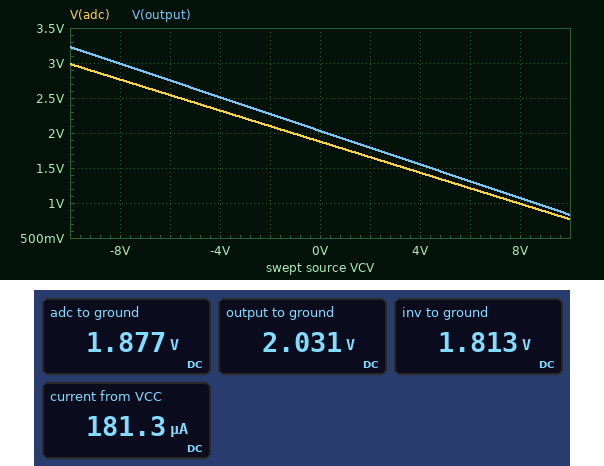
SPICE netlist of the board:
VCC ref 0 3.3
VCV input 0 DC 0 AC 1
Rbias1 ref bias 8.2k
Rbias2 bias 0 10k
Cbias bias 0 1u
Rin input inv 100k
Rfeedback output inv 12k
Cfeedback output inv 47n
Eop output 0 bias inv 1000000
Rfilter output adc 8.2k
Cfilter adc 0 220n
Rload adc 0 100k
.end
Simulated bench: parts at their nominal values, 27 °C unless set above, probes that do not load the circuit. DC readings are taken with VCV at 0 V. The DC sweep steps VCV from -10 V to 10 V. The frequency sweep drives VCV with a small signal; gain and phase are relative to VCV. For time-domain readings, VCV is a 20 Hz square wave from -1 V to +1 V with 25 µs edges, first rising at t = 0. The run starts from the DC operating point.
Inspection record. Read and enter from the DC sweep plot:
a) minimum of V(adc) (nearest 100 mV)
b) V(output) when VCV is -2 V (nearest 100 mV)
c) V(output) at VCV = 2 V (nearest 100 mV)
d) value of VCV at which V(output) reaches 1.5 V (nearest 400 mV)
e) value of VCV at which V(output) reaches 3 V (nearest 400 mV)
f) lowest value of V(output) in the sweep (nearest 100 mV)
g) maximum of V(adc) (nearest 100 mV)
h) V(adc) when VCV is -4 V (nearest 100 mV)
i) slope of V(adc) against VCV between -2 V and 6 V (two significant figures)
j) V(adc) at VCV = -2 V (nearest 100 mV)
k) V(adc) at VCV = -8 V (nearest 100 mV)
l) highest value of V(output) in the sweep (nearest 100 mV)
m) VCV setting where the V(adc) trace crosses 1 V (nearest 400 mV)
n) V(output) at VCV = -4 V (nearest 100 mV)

800 mV
2.3 V
1.8 V
4.4 V
-8.0 V
800 mV
3.0 V
2.3 V
-0.11 V/V
2.1 V
2.8 V
3.2 V
8.0 V
2.5 V
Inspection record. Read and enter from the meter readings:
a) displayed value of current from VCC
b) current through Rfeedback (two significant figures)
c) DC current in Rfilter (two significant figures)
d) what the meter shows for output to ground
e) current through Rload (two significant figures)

181.3 µA
18 µA
19 µA
2.031 V
19 µA
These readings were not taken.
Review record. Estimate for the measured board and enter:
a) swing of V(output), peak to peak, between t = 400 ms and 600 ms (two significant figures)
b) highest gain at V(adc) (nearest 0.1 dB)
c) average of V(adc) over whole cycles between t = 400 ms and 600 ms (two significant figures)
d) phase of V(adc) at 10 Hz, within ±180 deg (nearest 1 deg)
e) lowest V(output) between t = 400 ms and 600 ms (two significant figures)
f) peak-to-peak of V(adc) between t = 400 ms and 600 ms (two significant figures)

240 mV
-19.1 dB
1.9 V
172 deg
1.9 V
220 mV
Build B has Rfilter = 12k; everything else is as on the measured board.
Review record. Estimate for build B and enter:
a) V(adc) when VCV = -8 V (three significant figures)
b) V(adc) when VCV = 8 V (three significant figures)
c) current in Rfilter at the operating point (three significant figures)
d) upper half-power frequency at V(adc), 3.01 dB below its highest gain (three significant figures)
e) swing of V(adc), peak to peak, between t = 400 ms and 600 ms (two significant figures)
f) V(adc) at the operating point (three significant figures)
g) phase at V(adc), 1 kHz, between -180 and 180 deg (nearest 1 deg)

2.67 V
956 mV
18.1 µA
64.1 Hz
210 mV
1.81 V
20 deg
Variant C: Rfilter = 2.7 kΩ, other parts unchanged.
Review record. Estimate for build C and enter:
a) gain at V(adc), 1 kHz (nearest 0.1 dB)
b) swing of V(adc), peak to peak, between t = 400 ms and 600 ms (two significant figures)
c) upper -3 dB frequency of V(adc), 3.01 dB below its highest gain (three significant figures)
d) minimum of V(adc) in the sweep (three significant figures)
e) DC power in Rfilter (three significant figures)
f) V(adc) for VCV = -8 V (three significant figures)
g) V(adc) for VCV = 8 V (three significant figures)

-41.5 dB
230 mV
179 Hz
809 mV
1.06 µW
2.91 V
1.04 V
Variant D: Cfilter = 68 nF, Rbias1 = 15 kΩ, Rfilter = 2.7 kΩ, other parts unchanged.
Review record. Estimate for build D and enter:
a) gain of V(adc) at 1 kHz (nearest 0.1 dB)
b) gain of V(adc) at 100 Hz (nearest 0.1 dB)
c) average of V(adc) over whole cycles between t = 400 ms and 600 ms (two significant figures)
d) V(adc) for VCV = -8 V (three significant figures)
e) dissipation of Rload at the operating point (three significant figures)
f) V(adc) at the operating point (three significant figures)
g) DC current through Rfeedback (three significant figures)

-33.5 dB
-19.2 dB
1.4 V
2.37 V
20.7 µW
1.44 V
13.2 µA
